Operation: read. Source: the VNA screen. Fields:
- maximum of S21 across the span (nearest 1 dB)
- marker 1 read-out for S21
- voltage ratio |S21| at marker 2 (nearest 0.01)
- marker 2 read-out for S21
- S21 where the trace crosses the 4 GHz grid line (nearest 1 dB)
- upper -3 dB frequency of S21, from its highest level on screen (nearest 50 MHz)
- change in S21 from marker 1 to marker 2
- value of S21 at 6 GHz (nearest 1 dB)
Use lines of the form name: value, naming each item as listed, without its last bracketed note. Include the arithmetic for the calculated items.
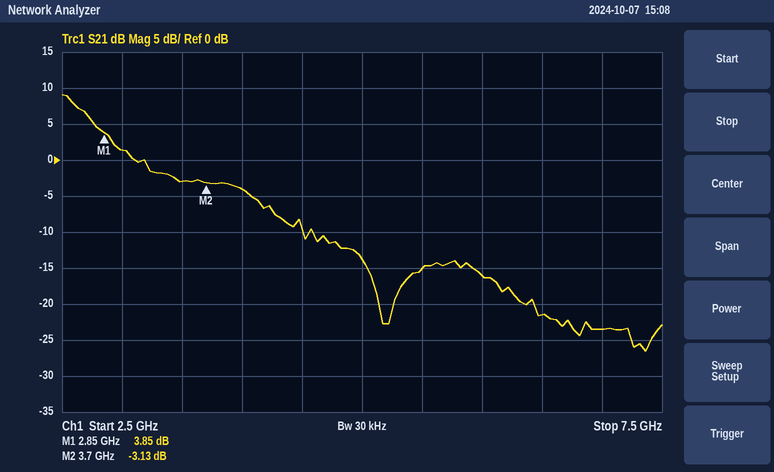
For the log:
maximum of S21 across the span: 9 dB
marker 1 read-out for S21: 3.85 dB
voltage ratio |S21| at marker 2: 10^(-3.13/20) ≈ 0.70
marker 2 read-out for S21: -3.13 dB
S21 where the trace crosses the 4 GHz grid line: -4 dB
upper -3 dB frequency of S21, from its highest level on screen: 2.70 GHz
change in S21 from marker 1 to marker 2: -3.13 − (3.85) = -6.98 dB
value of S21 at 6 GHz: -16 dB
